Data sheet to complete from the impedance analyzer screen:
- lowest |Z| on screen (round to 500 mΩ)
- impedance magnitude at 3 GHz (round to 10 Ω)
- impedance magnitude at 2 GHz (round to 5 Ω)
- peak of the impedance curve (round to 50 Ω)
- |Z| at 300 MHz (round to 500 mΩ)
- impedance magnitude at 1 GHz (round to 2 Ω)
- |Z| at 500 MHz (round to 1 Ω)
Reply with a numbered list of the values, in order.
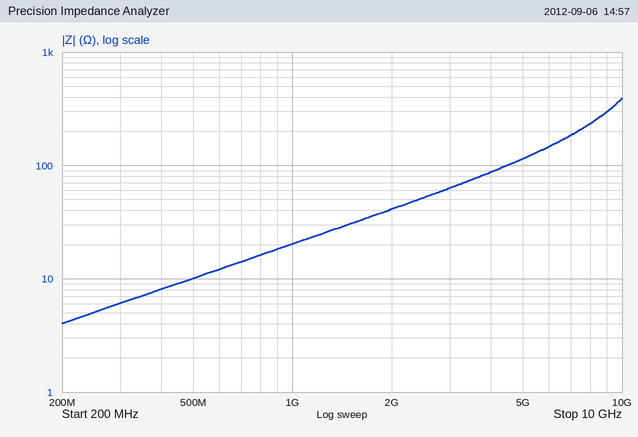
1. 4.0 Ω
2. 60 Ω
3. 40 Ω
4. 400 Ω
5. 6.0 Ω
6. 20 Ω
7. 10 Ω
